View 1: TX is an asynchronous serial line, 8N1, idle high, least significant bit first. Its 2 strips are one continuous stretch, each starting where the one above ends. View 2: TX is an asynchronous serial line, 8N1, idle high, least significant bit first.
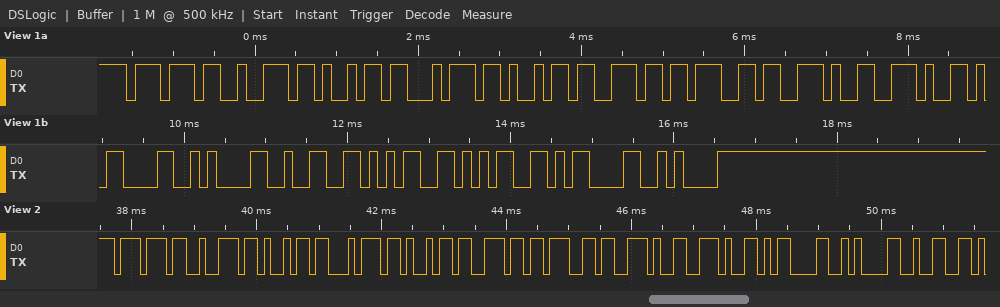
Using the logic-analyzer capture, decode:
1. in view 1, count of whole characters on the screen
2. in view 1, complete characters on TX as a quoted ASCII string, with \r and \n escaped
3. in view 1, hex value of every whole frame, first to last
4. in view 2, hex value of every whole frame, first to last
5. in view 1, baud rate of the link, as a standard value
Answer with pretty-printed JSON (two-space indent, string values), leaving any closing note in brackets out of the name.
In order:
{
  "in view 1, count of whole characters on the screen": "16",
  "in view 1, complete characters on TX as a quoted ASCII string, with \\r and \\n escaped": "\"writing..\\r\\n255\\r\\n\"",
  "in view 1, hex value of every whole frame, first to last": "77 72 69 74 69 6E 67 2E 2E 0D 0A 32 35 35 0D 0A",
  "in view 2, hex value of every whole frame, first to last": "77 72 69 74 69 6E 67 2E 2E 0D 0A 32",
  "in view 1, baud rate of the link, as a standard value": "9600 baud"
}
